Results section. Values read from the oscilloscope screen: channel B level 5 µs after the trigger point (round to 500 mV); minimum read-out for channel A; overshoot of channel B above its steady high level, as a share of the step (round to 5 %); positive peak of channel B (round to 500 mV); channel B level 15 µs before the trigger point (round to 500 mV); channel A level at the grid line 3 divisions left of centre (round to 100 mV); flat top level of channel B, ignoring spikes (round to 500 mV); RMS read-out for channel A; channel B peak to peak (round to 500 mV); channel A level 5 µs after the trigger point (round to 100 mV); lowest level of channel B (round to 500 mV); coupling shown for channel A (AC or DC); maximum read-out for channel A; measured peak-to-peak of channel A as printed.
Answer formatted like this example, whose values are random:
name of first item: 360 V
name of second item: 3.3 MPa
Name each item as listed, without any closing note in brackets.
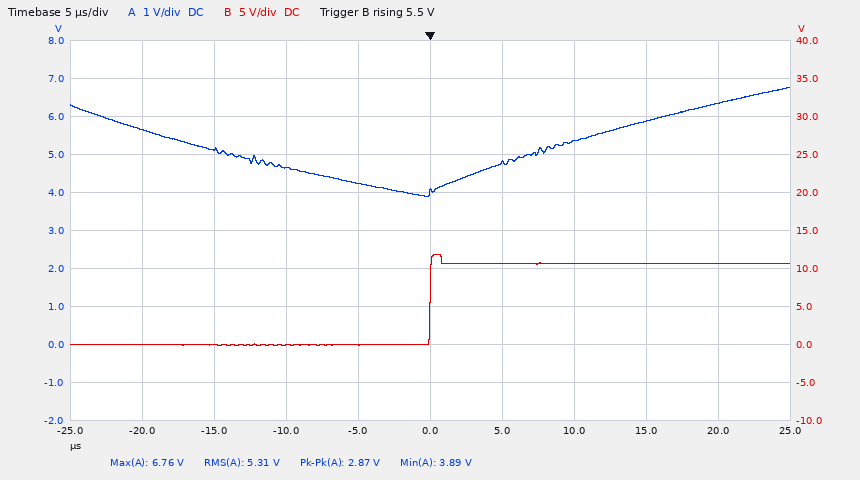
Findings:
channel B level 5 µs after the trigger point: 10.5 V
minimum read-out for channel A: 3.89 V
overshoot of channel B above its steady high level, as a share of the step: 10 %
positive peak of channel B: 12.0 V
channel B level 15 µs before the trigger point: 0.0 V
channel A level at the grid line 3 divisions left of centre: 5.1 V
flat top level of channel B, ignoring spikes: 10.5 V
RMS read-out for channel A: 5.31 V
channel B peak to peak: 12.0 V
channel A level 5 µs after the trigger point: 4.8 V
lowest level of channel B: 0.0 V
coupling shown for channel A: DC
maximum read-out for channel A: 6.76 V
measured peak-to-peak of channel A as printed: 2.87 V
